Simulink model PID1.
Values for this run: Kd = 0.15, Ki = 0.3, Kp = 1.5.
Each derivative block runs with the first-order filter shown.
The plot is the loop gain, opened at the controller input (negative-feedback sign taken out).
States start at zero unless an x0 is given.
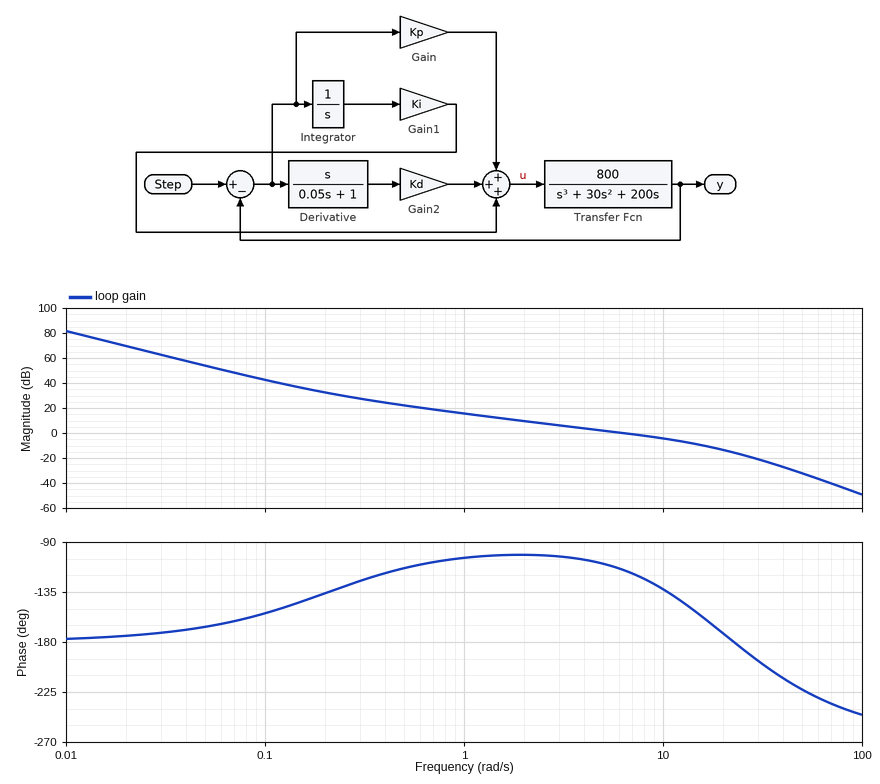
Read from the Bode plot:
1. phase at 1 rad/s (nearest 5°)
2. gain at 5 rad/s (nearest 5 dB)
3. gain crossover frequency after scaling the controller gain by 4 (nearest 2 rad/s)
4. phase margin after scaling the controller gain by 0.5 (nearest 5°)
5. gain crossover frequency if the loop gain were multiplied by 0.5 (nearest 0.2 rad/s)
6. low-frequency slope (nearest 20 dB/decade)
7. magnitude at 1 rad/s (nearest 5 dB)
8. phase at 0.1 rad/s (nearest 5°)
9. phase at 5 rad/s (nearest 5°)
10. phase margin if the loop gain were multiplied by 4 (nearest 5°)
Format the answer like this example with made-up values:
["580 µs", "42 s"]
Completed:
["-105°", "0 dB", "18 rad/s", "75°", "3.0 rad/s", "-40 dB/decade", "15 dB", "-155°", "-110°", "15°"]
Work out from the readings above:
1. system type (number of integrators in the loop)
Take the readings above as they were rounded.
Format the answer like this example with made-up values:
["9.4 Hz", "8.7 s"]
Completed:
["2"]
